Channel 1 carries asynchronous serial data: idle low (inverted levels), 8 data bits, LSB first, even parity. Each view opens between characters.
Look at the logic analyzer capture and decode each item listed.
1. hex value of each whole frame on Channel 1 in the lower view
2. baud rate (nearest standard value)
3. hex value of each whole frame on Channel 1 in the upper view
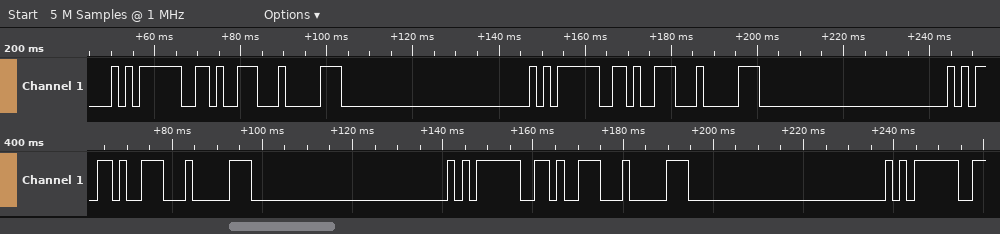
1A, 1F, 05, 1A, 1F, 05
600 baud
05, 1A, 1F, 05, 1A, 1F
